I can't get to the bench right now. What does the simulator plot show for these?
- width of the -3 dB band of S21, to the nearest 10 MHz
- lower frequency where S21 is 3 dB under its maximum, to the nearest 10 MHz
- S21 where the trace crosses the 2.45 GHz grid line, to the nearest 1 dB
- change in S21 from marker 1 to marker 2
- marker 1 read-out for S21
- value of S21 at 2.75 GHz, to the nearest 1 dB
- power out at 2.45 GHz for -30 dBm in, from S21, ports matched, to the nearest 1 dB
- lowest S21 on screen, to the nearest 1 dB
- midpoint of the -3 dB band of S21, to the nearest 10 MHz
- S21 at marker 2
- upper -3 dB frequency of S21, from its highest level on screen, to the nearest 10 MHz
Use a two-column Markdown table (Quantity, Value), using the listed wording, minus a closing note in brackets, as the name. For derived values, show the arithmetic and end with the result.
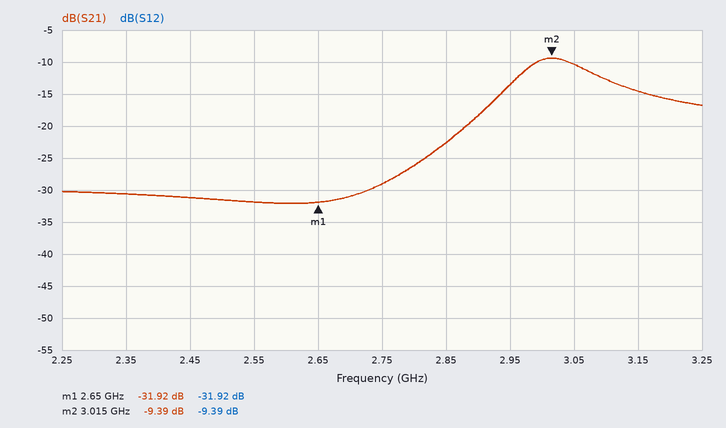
| Quantity | Value |
|---|---|
| width of the -3 dB band of S21, to the nearest 10 MHz | 3.09 GHz − 2.96 GHz = 130 MHz |
| lower frequency where S21 is 3 dB under its maximum, to the nearest 10 MHz | 2.96 GHz |
| S21 where the trace crosses the 2.45 GHz grid line, to the nearest 1 dB | -31 dB |
| change in S21 from marker 1 to marker 2 | -9.39 − (-31.92) = 22.53 dB |
| marker 1 read-out for S21 | -31.92 dB |
| value of S21 at 2.75 GHz, to the nearest 1 dB | -29 dB |
| power out at 2.45 GHz for -30 dBm in, from S21, ports matched, to the nearest 1 dB | -30 dBm + (-31 dB) = -61 dBm |
| lowest S21 on screen, to the nearest 1 dB | -32 dB |
| midpoint of the -3 dB band of S21, to the nearest 10 MHz | 3.03 GHz |
| S21 at marker 2 | -9.39 dB |
| upper -3 dB frequency of S21, from its highest level on screen, to the nearest 10 MHz | 3.09 GHz |
